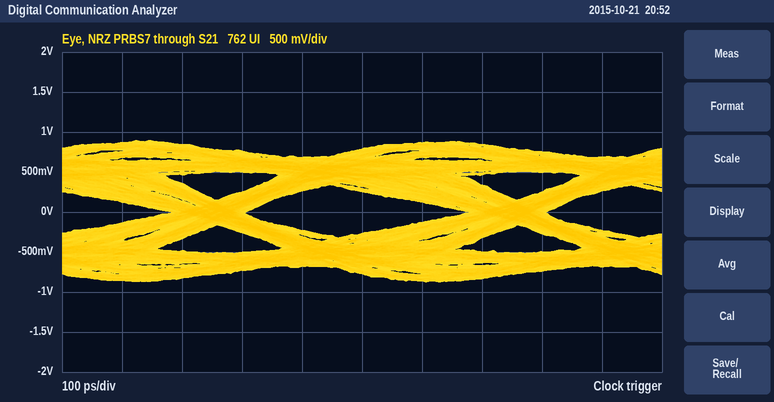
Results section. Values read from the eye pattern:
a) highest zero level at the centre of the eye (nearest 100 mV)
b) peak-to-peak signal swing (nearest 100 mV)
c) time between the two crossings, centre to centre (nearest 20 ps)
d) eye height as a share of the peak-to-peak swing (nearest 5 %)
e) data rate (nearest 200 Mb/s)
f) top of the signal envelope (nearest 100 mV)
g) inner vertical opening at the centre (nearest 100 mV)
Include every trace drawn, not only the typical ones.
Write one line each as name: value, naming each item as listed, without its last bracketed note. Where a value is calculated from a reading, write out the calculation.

highest zero level at the centre of the eye: -300 mV
peak-to-peak signal swing: 1.8 V
time between the two crossings, centre to centre: 500 ps
eye height as a share of the peak-to-peak swing: 500 mV / 1.8 V ≈ 27.8 %, so 30 % to the nearest 5 %
data rate: 2.0 Gb/s
top of the signal envelope: 900 mV
inner vertical opening at the centre: 500 mV
